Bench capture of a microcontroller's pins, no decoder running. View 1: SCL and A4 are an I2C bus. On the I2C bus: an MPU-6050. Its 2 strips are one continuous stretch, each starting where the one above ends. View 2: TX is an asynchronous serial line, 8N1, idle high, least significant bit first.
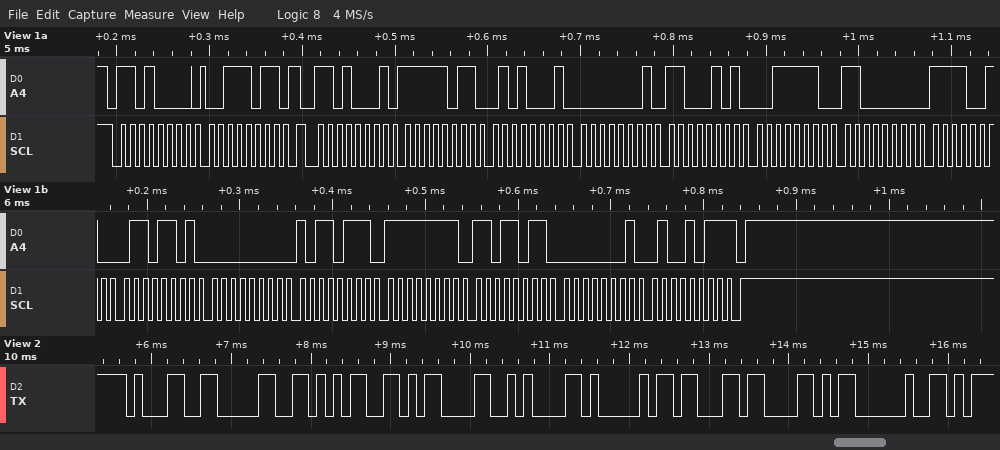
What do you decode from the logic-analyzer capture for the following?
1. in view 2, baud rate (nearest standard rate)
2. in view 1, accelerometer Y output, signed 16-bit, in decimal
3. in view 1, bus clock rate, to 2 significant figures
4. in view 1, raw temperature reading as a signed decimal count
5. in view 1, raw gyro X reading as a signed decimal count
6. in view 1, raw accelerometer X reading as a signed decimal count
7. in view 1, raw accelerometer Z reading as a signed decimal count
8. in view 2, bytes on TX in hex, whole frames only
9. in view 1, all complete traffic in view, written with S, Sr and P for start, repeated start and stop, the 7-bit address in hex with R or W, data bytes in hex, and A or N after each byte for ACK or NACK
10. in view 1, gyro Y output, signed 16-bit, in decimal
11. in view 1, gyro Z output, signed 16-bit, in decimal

9600 baud
453
100 kHz
-3475
183
-1199
16064
31 30 35 0D 0A 41 63 58 20
S 68W A 3B A Sr 68R A FB A 51 A 01 A C5 A 3E A C0 A F2 A 6D A 00 A B7 A FF A DB A 01 A 4B N P
-37
331
